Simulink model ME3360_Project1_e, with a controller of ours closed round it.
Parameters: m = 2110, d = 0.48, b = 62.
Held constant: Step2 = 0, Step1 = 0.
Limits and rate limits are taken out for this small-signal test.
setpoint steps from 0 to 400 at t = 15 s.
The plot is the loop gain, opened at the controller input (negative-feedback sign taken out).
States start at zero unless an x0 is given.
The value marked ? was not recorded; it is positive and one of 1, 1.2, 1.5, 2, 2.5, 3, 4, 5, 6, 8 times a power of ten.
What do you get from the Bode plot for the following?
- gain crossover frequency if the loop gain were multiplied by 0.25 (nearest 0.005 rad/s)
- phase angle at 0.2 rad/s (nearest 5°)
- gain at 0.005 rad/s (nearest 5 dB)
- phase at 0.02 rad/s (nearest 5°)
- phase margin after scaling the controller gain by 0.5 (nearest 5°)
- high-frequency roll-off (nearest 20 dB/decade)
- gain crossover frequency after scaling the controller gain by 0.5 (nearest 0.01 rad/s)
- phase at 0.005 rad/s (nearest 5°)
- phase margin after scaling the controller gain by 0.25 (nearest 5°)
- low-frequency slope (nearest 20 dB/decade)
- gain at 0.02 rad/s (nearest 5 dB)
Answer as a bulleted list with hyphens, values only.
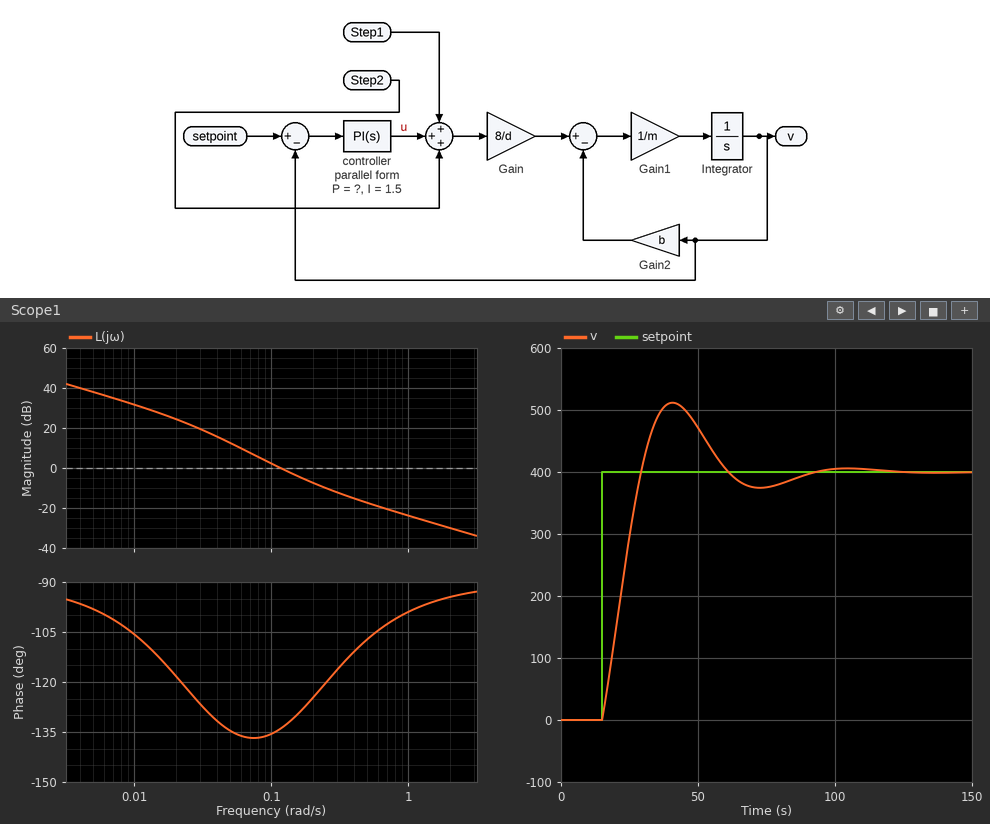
- 0.050 rad/s
- -125°
- 40 dB
- -120°
- 45°
- -20 dB/decade
- 0.08 rad/s
- -100°
- 45°
- -20 dB/decade
- 25 dB
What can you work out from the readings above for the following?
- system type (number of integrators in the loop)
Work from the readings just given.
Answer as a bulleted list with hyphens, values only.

- 1
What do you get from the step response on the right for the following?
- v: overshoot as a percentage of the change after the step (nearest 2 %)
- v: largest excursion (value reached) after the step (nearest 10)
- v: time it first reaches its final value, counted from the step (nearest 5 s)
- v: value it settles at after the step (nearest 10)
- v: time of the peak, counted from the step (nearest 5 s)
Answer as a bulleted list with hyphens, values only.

- 28 %
- 510
- 15 s
- 400
- 25 s
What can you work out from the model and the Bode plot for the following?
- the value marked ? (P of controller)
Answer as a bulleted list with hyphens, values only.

- 8
